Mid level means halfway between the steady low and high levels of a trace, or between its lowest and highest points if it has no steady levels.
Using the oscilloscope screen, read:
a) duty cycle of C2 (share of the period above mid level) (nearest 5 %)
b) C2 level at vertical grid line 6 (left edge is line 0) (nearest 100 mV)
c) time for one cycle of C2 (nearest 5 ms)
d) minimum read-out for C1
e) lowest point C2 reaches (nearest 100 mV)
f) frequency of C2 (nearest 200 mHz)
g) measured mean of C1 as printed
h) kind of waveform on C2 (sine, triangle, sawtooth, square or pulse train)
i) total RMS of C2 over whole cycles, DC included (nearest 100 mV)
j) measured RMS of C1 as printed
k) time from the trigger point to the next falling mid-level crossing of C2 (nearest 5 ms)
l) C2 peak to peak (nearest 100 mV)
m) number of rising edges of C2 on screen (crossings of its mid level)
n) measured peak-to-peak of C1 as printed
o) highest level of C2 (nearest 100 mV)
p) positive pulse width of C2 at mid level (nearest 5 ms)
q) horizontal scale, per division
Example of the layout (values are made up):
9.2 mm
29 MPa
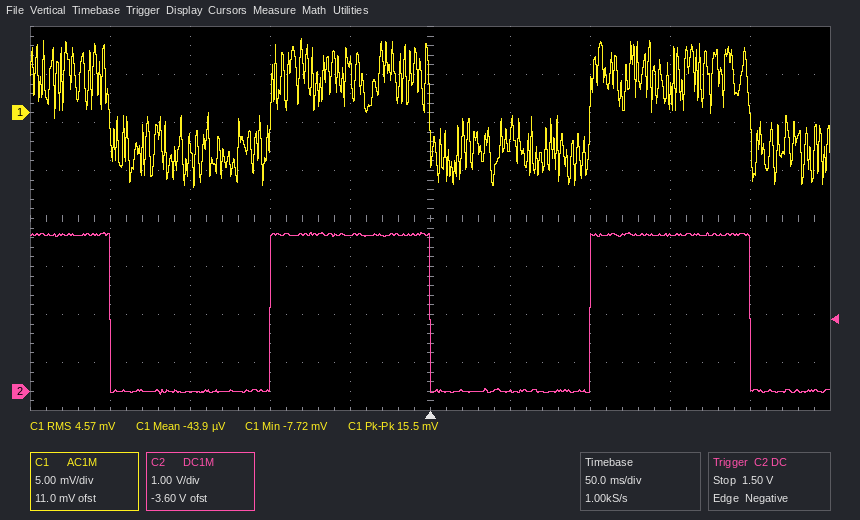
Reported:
50 %
0.0 V
200 ms
-7.72 mV
-100 mV
5.0 Hz
-43.9 µV
square
2.3 V
4.57 mV
200 ms
3.4 V
2
15.5 mV
3.3 V
100 ms
50 ms
